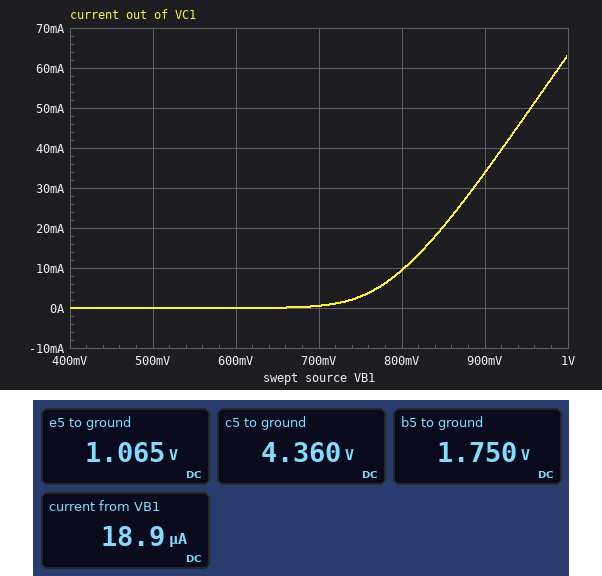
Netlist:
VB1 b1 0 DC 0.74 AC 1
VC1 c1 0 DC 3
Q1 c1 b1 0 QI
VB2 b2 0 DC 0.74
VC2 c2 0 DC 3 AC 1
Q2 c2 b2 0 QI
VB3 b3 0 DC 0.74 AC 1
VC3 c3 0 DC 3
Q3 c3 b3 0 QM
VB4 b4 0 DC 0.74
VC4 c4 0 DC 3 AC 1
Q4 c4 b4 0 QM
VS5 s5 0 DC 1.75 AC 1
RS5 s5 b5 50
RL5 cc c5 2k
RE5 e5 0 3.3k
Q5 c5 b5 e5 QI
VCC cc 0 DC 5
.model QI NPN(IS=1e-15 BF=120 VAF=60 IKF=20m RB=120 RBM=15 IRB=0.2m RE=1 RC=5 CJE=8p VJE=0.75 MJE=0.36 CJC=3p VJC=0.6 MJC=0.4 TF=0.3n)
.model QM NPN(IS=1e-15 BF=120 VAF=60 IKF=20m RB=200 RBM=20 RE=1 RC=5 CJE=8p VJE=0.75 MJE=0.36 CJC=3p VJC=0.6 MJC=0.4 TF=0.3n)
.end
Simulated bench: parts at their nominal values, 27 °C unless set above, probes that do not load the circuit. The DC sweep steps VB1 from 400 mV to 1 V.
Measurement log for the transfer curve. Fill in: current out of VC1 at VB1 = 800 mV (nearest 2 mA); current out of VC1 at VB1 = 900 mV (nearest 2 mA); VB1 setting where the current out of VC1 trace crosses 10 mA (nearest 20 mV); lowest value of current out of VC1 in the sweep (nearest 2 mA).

10 mA
34 mA
800 mV
0 A
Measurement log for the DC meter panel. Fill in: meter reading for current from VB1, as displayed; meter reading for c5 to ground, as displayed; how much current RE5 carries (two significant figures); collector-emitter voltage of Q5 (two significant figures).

18.9 µA
4.360 V
320 µA
3.3 V
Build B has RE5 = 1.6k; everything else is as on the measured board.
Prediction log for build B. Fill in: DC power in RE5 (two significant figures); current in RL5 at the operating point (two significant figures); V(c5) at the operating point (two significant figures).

680 µW
650 µA
3.7 V
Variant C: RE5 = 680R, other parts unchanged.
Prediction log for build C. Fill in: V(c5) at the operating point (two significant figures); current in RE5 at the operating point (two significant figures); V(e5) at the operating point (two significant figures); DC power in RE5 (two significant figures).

2.0 V
1.5 mA
1.0 V
1.5 mW
